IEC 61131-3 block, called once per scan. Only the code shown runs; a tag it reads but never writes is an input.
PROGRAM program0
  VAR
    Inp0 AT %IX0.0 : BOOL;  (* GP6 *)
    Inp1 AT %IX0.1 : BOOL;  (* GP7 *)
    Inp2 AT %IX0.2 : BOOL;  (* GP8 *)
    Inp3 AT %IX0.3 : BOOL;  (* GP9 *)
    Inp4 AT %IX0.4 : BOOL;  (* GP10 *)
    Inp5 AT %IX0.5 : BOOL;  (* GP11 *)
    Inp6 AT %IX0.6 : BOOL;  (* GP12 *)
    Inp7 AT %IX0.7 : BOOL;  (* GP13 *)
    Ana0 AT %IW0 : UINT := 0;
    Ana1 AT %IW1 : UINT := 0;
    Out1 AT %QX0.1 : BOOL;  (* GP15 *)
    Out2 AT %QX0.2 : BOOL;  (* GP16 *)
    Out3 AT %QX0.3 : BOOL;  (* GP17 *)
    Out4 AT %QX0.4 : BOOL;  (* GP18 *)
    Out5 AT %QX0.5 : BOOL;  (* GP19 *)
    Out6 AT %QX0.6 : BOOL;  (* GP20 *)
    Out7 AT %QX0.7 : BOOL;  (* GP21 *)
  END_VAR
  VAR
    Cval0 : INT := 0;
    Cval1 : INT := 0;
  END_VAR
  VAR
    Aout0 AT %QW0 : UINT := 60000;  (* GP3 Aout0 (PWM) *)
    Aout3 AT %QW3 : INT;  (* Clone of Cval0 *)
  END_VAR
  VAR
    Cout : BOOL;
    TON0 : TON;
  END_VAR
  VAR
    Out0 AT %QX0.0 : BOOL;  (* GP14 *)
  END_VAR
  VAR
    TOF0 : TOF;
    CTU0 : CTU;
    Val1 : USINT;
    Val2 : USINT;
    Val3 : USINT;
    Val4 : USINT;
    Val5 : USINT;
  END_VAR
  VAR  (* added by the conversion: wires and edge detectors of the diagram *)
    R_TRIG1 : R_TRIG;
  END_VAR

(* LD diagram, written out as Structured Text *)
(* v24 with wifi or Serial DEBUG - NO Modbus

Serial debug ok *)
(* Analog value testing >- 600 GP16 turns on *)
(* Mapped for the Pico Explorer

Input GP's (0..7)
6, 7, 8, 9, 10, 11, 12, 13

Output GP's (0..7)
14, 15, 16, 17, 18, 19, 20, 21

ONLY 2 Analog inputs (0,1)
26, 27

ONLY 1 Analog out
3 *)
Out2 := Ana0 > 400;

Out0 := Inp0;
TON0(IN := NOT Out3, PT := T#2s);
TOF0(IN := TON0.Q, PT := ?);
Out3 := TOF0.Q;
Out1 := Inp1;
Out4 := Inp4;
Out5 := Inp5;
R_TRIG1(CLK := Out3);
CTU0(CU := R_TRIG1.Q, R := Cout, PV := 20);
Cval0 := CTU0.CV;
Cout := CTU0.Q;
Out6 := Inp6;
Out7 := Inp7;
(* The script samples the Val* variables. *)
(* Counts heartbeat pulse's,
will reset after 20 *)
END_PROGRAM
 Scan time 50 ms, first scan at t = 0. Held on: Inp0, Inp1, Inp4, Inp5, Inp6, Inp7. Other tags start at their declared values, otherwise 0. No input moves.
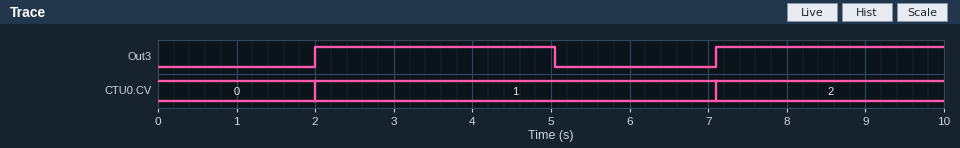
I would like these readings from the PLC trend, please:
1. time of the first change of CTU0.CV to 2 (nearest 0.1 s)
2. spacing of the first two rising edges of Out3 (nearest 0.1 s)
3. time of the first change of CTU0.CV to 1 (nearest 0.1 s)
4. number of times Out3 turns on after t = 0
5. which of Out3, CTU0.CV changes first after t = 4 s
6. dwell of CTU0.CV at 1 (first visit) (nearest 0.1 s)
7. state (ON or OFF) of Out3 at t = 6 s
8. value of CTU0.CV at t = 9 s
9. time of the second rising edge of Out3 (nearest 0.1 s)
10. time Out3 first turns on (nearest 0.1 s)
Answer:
7.1 s
5.1 s
2.0 s
2
Out3
5.1 s
OFF
2
7.1 s
2.0 s
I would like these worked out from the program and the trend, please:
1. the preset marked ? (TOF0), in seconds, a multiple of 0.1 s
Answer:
3.0 s
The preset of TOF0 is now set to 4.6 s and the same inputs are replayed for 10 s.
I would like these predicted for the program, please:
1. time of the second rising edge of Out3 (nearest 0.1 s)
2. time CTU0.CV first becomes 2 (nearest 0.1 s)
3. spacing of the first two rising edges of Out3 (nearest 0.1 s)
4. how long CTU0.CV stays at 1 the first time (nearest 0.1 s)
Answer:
8.7 s
8.7 s
6.7 s
6.7 s
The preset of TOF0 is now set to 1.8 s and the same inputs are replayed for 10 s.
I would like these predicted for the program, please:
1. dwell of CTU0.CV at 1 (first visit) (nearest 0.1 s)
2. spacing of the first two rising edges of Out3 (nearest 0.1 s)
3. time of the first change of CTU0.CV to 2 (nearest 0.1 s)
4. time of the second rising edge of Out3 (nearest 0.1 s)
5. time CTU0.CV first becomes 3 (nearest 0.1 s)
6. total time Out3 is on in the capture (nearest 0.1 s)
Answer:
3.9 s
3.9 s
5.9 s
5.9 s
9.8 s
3.9 s
